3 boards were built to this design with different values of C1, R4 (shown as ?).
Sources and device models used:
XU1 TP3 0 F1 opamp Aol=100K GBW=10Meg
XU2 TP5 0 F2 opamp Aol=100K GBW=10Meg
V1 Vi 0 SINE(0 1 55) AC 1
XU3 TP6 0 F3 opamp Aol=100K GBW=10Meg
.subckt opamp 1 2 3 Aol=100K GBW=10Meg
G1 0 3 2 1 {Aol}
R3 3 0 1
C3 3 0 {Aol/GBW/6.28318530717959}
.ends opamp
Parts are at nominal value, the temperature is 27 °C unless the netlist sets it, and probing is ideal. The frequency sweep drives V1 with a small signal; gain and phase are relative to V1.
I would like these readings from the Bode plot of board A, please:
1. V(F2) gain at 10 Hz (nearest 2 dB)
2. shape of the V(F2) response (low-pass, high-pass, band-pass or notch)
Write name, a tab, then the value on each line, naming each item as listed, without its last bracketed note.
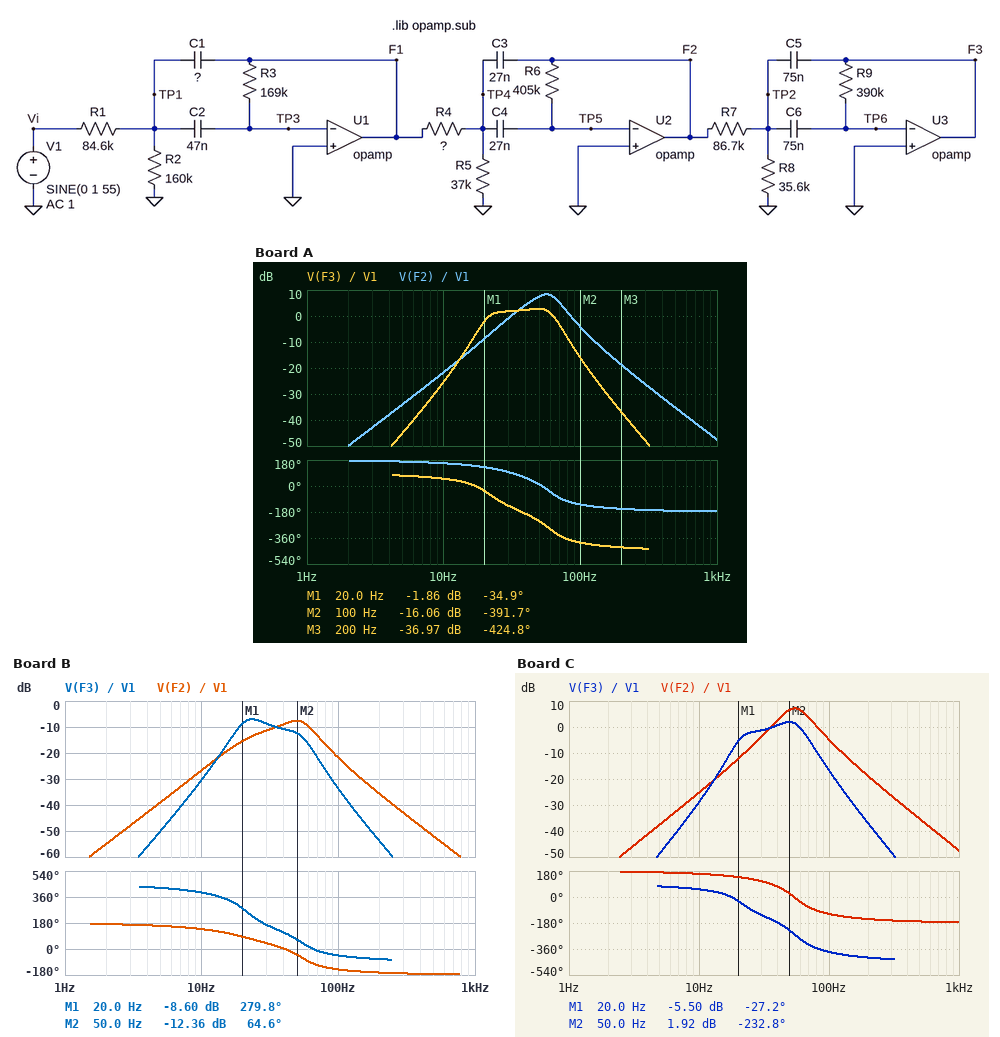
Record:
V(F2) gain at 10 Hz	-22 dB
shape of the V(F2) response	band-pass
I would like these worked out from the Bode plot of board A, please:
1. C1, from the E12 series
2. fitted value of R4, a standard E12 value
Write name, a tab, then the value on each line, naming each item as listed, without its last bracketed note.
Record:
C1, from the E12 series	39 nF
fitted value of R4, a standard E12 value	68 kΩ
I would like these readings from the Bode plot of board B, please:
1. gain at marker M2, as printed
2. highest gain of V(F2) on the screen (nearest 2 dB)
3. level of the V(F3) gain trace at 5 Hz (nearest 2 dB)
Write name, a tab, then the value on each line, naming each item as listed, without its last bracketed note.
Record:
gain at marker M2, as printed	-12.36 dB
highest gain of V(F2) on the screen	-8 dB
level of the V(F3) gain trace at 5 Hz	-50 dB
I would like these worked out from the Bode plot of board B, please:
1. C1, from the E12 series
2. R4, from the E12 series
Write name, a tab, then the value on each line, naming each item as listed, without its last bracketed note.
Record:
C1, from the E12 series	120 nF
R4, from the E12 series	150 kΩ
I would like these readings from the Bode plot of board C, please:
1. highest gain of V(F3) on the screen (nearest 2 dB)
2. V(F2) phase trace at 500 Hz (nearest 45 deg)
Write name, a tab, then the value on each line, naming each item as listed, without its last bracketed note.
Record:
highest gain of V(F3) on the screen	2 dB
V(F2) phase trace at 500 Hz	-180 deg
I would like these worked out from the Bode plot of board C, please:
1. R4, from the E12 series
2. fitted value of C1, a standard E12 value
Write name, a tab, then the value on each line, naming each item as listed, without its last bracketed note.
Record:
R4, from the E12 series	120 kΩ
fitted value of C1, a standard E12 value	22 nF
